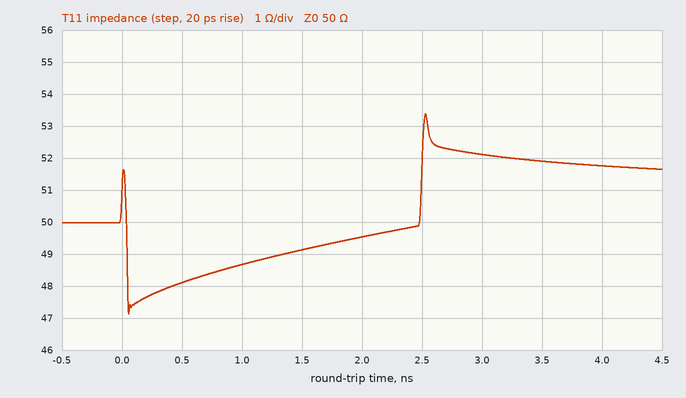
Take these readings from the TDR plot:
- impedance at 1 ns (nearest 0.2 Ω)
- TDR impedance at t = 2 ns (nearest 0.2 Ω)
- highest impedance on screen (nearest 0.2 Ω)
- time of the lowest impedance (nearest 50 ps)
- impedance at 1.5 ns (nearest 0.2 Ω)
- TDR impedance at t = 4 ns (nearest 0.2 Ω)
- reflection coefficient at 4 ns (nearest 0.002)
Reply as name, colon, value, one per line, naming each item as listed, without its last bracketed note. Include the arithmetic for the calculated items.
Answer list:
impedance at 1 ns: 48.6 Ω
TDR impedance at t = 2 ns: 49.6 Ω
highest impedance on screen: 53.4 Ω
time of the lowest impedance: 50 ps
impedance at 1.5 ns: 49.2 Ω
TDR impedance at t = 4 ns: 51.8 Ω
reflection coefficient at 4 ns: (51.8 − 50)/(51.8 + 50) ≈ +0.018
